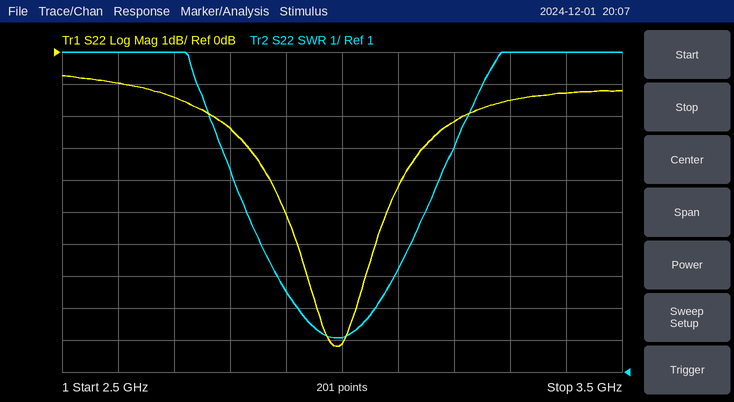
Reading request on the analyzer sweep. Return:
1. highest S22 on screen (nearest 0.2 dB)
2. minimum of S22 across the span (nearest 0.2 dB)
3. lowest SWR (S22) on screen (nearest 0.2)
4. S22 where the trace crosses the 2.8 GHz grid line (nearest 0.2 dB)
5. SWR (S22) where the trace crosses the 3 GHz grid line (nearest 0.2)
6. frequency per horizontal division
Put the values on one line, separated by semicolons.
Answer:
-0.8 dB; -9.2 dB; 2.0; -2.4 dB; 2.0; 100 MHz
